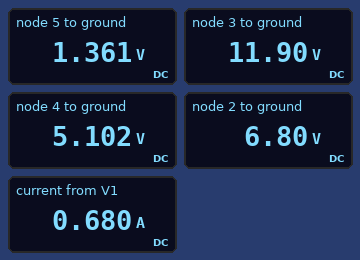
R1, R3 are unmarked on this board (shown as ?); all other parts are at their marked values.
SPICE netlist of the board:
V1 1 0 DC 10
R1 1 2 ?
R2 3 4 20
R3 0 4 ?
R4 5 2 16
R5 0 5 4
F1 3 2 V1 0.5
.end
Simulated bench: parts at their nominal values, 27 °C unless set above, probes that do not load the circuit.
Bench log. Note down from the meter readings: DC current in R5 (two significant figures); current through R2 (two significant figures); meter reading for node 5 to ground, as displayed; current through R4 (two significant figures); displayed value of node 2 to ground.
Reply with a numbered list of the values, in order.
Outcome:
1. 340 mA
2. 340 mA
3. 1.361 V
4. 340 mA
5. 6.80 V
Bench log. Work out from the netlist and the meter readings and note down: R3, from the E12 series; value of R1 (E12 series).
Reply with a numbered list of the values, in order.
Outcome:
1. 15 Ω
2. 4.7 Ω
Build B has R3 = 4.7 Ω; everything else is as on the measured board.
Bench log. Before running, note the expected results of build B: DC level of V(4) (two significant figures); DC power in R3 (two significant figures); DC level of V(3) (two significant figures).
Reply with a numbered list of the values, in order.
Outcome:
1. 1.6 V
2. 540 mW
3. 8.4 V
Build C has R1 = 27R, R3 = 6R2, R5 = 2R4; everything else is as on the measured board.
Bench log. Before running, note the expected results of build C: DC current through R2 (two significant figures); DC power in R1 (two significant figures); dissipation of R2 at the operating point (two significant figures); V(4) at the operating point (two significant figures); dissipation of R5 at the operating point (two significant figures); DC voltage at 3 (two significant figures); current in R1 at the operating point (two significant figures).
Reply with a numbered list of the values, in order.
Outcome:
1. 140 mA
2. 2.1 W
3. 380 mW
4. 860 mV
5. 46 mW
6. 3.6 V
7. 280 mA
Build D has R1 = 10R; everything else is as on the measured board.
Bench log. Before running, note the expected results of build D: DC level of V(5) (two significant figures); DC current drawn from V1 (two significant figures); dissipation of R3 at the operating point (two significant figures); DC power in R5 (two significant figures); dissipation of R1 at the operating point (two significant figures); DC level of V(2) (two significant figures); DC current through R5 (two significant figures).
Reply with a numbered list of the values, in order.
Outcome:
1. 1.0 V
2. 500 mA
3. 940 mW
4. 250 mW
5. 2.5 W
6. 5.0 V
7. 250 mA
